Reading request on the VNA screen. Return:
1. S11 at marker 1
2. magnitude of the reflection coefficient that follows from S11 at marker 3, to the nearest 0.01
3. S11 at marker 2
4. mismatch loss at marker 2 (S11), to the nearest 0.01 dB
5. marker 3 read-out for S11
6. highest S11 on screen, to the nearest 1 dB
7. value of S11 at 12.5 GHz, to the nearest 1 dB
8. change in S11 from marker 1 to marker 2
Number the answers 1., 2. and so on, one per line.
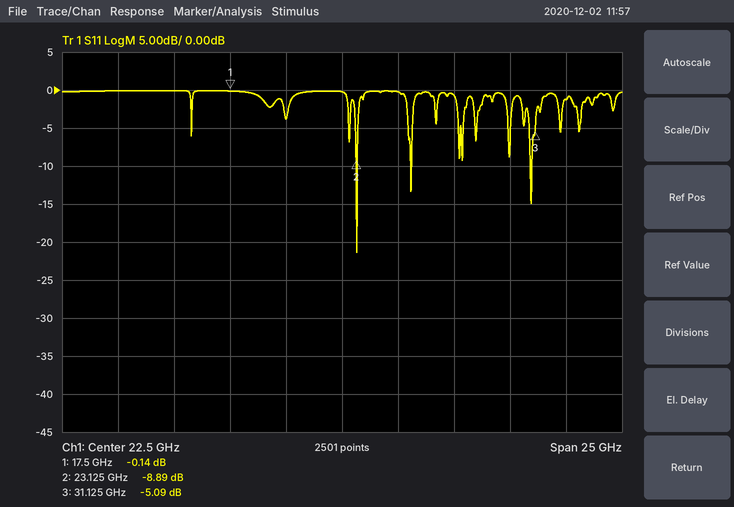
1. -0.14 dB
2. 0.56
3. -8.89 dB
4. 0.60 dB
5. -5.09 dB
6. 0 dB
7. 0 dB
8. -8.75 dB
